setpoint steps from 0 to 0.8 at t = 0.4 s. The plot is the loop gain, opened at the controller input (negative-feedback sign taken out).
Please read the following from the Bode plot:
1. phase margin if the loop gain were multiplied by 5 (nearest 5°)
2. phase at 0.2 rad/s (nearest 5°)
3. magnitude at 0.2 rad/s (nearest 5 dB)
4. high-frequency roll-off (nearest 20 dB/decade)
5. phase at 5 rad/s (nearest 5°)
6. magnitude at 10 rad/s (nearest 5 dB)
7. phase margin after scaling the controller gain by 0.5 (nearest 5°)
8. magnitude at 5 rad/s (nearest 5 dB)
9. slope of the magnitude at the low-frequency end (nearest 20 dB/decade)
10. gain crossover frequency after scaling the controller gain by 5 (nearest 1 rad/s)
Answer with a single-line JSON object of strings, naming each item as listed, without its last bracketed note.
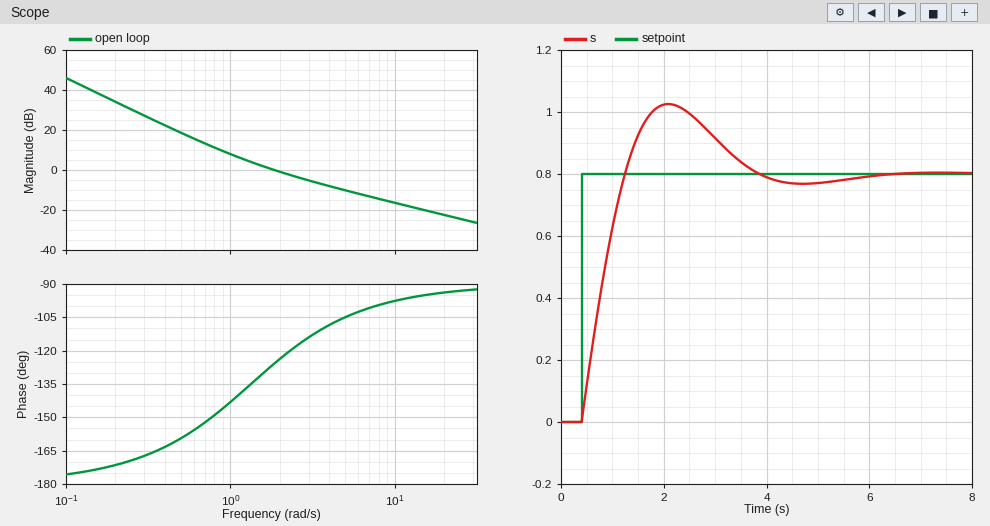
{"phase margin if the loop gain were multiplied by 5": "80°", "phase at 0.2 rad/s": "-170°", "magnitude at 0.2 rad/s": "35 dB", "high-frequency roll-off": "-20 dB/decade", "phase at 5 rad/s": "-105°", "magnitude at 10 rad/s": "-15 dB", "phase margin after scaling the controller gain by 0.5": "40°", "magnitude at 5 rad/s": "-10 dB", "slope of the magnitude at the low-frequency end": "-40 dB/decade", "gain crossover frequency after scaling the controller gain by 5": "8 rad/s"}
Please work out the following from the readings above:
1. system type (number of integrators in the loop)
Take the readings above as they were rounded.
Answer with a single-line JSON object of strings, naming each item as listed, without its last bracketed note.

{"system type": "2"}
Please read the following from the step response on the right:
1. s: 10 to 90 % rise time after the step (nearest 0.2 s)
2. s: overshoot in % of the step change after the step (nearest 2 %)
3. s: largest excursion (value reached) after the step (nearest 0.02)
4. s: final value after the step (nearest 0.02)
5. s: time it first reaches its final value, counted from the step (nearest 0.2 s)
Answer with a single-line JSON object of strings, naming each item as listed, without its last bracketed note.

{"s: 10 to 90 % rise time after the step": "0.6 s", "s: overshoot in % of the step change after the step": "28 %", "s: largest excursion (value reached) after the step": "1.02", "s: final value after the step": "0.80", "s: time it first reaches its final value, counted from the step": "0.8 s"}
